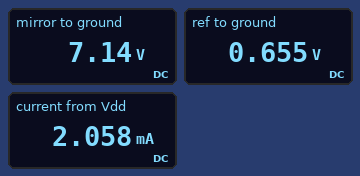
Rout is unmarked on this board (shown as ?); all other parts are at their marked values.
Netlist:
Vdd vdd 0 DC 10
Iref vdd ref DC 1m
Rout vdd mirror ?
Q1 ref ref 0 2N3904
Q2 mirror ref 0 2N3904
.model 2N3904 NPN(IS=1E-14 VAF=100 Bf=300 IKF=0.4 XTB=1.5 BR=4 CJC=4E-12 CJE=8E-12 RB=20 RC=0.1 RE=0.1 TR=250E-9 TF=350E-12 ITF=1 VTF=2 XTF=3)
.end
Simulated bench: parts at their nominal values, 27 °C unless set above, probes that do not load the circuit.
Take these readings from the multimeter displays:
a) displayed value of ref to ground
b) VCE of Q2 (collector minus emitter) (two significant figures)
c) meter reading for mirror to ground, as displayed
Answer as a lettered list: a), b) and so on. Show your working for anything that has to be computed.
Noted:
a) 0.655 V
b) 7.14 V = 7.1 V
c) 7.14 V
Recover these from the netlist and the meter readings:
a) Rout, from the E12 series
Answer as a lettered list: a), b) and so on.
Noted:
a) 2.7 kΩ
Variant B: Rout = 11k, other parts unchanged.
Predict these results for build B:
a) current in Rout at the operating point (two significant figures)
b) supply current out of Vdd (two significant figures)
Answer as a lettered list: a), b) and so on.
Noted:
a) 900 µA
b) 1.9 mA
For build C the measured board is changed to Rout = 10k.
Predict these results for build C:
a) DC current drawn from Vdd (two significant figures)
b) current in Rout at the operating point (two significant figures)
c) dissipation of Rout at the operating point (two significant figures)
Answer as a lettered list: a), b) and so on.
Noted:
a) 2.0 mA
b) 980 µA
c) 9.7 mW
